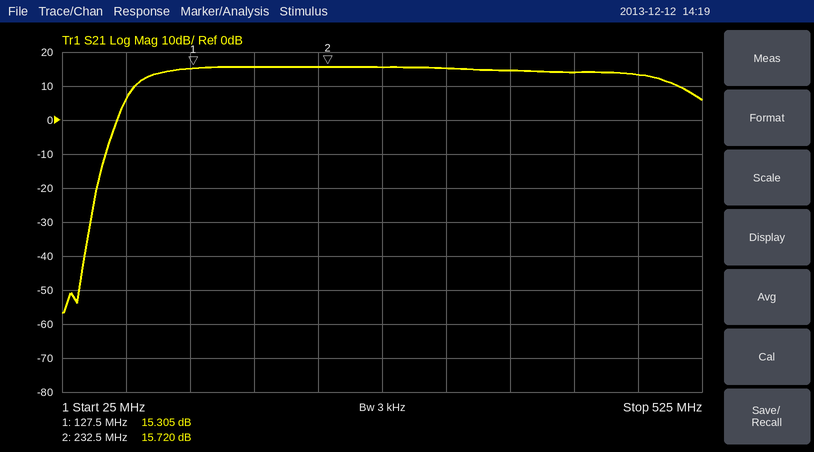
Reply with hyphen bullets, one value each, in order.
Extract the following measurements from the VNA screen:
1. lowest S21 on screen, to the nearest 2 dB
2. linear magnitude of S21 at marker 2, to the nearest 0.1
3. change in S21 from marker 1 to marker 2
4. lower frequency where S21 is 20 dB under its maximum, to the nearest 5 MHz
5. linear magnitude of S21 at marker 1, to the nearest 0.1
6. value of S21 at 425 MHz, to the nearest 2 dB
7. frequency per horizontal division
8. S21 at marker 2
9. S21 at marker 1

- -56 dB
- 6.1
- 0.415 dB
- 65 MHz
- 5.8
- 14 dB
- 50 MHz
- 15.720 dB
- 15.305 dB
